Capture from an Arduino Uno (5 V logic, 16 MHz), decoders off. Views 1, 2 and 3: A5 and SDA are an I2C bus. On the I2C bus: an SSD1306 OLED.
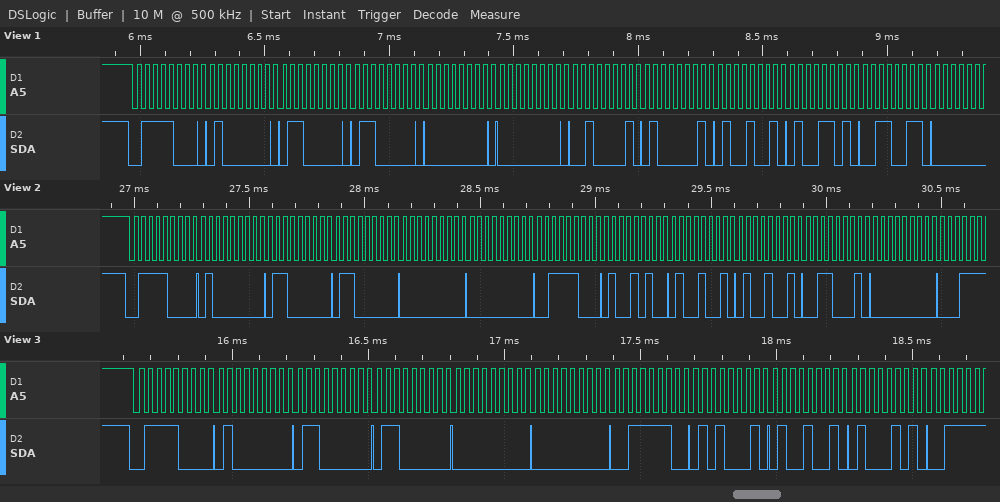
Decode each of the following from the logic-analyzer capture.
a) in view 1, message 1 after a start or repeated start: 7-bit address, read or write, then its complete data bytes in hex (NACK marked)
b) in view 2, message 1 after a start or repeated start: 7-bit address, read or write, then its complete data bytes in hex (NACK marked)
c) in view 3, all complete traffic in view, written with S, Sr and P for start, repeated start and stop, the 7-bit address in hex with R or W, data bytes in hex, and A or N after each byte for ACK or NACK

0x3C write: 40 60 60 00 00 21 41 49 4D 33
0x3C write: 40 60 60 00 00 3C 4A 49 49 31 00
S 3CW A 40 A 60 A 60 A 00 A 00 A 3E A 51 A 49 A 45 A
